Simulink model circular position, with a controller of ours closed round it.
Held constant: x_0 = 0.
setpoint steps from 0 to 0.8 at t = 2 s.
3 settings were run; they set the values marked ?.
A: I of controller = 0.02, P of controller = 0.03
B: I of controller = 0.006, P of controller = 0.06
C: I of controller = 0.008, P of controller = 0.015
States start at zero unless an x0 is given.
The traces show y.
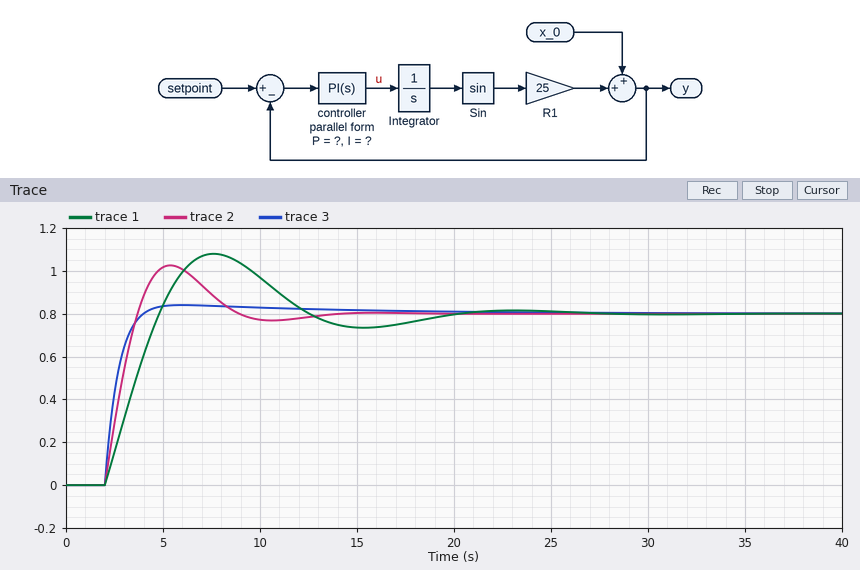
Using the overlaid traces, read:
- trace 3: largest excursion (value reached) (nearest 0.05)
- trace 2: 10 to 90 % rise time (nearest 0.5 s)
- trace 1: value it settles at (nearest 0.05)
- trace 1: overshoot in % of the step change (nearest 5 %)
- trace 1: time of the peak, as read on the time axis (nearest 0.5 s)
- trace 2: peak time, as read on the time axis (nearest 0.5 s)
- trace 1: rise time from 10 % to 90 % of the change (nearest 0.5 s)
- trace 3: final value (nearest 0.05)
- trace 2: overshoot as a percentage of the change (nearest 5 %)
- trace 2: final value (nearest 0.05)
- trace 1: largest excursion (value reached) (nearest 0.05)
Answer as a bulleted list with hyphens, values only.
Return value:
- 0.85
- 1.5 s
- 0.80
- 35 %
- 7.5 s
- 5.5 s
- 2.0 s
- 0.80
- 30 %
- 0.80
- 1.10
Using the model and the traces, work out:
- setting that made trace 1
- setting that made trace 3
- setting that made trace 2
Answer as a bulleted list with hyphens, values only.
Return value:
- C
- B
- A
